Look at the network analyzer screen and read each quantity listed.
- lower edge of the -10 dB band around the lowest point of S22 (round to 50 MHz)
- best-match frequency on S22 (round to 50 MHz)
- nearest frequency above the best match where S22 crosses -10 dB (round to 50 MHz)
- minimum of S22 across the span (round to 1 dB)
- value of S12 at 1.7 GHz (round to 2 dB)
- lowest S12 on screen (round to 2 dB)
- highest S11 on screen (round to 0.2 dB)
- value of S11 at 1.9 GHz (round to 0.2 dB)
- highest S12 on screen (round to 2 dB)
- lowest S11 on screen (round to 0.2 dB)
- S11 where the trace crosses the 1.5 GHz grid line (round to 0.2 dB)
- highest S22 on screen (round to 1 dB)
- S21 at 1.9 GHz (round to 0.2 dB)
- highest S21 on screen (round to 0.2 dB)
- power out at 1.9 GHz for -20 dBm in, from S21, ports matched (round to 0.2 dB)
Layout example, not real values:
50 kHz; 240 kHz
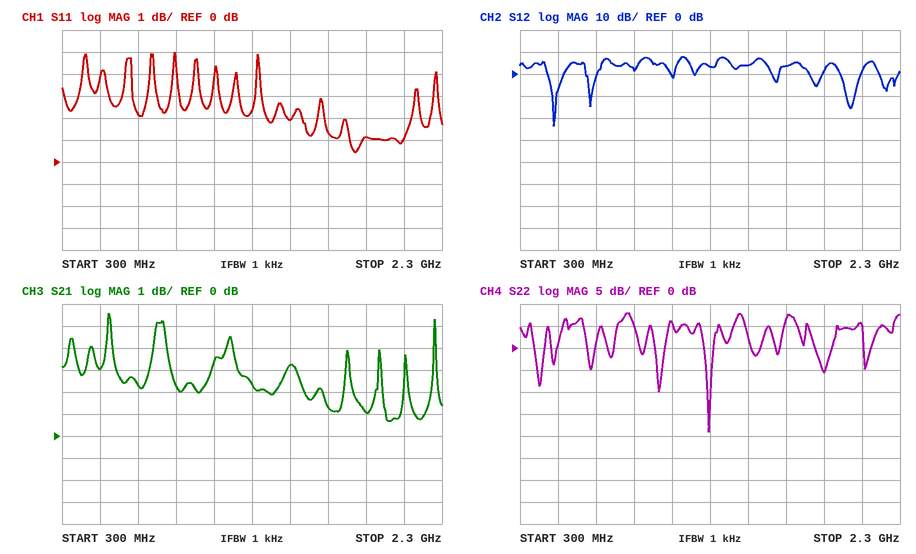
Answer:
1.30 GHz; 1.30 GHz; 1.30 GHz; -19 dB; 4 dB; -24 dB; 5.0 dB; 1.2 dB; 8 dB; 0.4 dB; 2.0 dB; 8 dB; 1.0 dB; 5.6 dB; -19.0 dBm
